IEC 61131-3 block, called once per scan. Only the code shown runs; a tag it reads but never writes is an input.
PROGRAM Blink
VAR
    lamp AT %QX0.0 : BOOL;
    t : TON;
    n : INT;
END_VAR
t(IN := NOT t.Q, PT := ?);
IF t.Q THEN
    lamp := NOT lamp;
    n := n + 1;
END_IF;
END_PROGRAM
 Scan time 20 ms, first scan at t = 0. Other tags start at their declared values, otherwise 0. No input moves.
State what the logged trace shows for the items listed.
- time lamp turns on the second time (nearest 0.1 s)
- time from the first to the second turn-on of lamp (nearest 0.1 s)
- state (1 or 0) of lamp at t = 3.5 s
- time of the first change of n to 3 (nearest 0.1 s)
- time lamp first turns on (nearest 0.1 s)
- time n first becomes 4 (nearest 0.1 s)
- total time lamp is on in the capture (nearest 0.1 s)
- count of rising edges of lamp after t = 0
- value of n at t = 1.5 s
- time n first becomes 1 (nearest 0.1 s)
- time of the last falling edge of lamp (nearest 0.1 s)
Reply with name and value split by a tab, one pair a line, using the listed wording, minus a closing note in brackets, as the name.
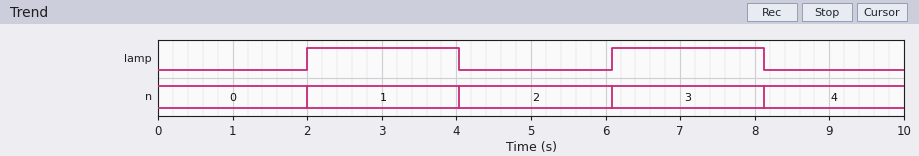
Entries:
time lamp turns on the second time	6.1 s
time from the first to the second turn-on of lamp	4.1 s
state (1 or 0) of lamp at t = 3.5 s	1
time of the first change of n to 3	6.1 s
time lamp first turns on	2.0 s
time n first becomes 4	8.1 s
total time lamp is on in the capture	4.1 s
count of rising edges of lamp after t = 0	2
value of n at t = 1.5 s	0
time n first becomes 1	2.0 s
time of the last falling edge of lamp	8.1 s
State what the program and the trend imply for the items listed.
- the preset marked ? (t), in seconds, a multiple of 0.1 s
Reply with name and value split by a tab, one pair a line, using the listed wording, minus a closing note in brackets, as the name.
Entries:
the preset marked ? (t), in seconds, a multiple of 0.1 s	2.0 s
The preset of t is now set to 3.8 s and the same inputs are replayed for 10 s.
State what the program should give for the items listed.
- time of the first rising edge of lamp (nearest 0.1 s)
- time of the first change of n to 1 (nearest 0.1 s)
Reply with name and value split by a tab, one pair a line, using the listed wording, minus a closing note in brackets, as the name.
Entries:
time of the first rising edge of lamp	3.8 s
time of the first change of n to 1	3.8 s
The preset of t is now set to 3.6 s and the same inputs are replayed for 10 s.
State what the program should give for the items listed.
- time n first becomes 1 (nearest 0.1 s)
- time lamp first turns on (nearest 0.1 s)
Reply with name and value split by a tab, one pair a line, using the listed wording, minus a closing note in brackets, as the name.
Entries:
time n first becomes 1	3.6 s
time lamp first turns on	3.6 s
